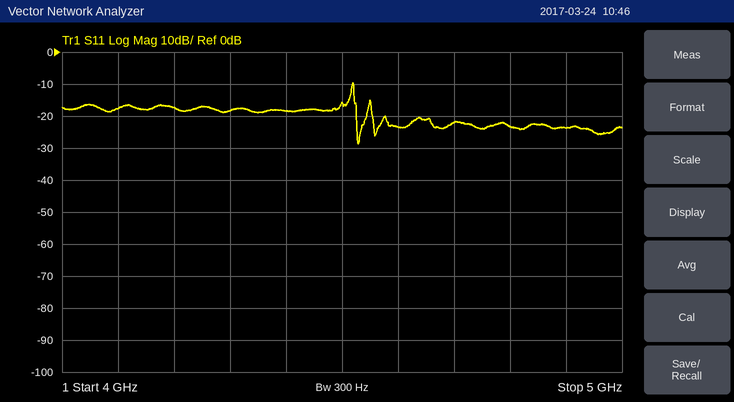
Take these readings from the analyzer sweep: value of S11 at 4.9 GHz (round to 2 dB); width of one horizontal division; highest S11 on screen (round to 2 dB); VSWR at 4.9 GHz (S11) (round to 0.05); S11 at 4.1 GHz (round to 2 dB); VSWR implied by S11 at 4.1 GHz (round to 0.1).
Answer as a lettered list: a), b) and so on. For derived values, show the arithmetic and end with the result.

a) -24 dB
b) 100 MHz
c) -10 dB
d) |Γ| = 10^(-24/20) = 0.0631; VSWR = (1 + 0.0631)/(1 − 0.0631) ≈ 1.13, so 1.15 to the nearest 0.05
e) -18 dB
f) |Γ| = 10^(-18/20) = 0.1259; VSWR = (1 + 0.1259)/(1 − 0.1259) ≈ 1.3
